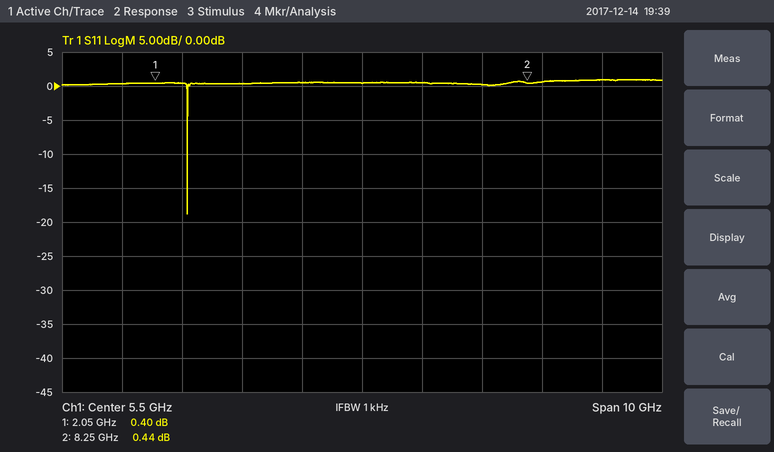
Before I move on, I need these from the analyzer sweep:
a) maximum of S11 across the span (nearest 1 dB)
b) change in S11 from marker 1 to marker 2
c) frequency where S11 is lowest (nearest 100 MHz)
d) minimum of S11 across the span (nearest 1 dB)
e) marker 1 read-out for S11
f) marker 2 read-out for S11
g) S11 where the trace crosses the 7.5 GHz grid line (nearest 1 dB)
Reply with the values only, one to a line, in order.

1 dB
0.04 dB
2.6 GHz
-19 dB
0.40 dB
0.44 dB
0 dB
